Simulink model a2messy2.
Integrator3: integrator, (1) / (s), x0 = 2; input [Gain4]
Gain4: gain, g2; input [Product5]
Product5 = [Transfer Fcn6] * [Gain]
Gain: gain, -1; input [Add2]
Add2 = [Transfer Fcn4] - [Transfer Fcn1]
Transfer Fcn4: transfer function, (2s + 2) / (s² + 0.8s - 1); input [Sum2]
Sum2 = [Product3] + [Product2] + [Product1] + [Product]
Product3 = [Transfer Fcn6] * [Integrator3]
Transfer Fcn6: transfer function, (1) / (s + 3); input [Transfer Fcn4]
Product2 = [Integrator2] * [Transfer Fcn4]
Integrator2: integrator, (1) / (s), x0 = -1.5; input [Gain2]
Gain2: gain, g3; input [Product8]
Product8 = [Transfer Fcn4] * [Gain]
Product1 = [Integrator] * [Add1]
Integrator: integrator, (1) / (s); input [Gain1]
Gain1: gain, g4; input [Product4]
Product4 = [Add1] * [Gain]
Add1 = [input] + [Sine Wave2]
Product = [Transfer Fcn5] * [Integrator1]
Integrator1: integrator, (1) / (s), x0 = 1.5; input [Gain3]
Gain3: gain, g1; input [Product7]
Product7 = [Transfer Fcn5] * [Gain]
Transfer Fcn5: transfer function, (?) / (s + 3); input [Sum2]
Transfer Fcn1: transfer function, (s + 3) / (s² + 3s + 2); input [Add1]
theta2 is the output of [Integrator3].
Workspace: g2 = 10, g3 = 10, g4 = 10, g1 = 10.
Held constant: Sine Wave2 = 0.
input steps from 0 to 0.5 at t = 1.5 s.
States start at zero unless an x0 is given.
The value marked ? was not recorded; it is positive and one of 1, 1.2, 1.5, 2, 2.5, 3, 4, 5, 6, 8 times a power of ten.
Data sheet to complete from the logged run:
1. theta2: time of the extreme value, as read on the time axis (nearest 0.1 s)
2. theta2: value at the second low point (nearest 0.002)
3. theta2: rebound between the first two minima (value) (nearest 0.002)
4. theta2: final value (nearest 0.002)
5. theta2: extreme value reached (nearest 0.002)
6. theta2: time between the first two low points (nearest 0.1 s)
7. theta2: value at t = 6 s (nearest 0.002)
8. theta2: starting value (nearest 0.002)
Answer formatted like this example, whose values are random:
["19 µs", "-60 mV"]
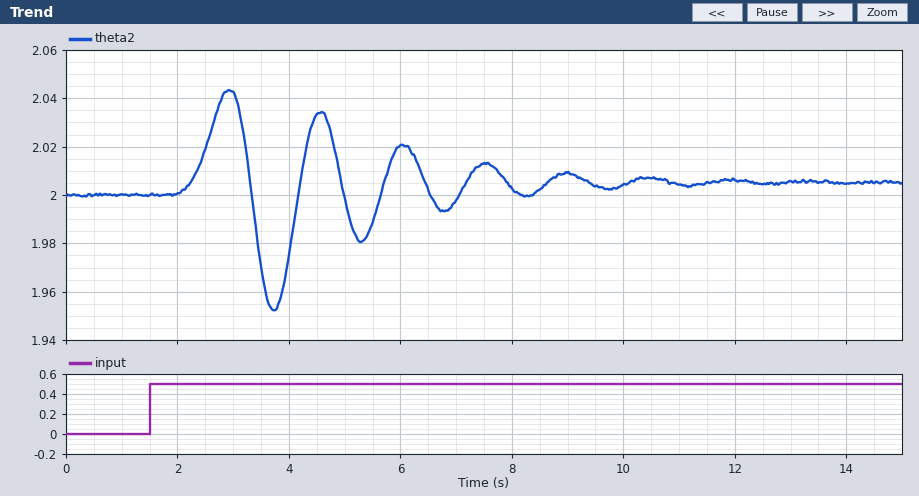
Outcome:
["3.7 s", "1.980", "2.034", "2.006", "1.952", "1.6 s", "2.020", "2.000"]
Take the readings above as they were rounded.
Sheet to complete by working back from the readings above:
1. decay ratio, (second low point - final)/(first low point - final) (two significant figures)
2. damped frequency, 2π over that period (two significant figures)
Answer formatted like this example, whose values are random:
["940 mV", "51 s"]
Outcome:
["0.48", "3.9 rad/s"]
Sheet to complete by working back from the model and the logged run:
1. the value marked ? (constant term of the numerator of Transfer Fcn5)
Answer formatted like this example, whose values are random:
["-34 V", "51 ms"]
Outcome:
["1.2"]
